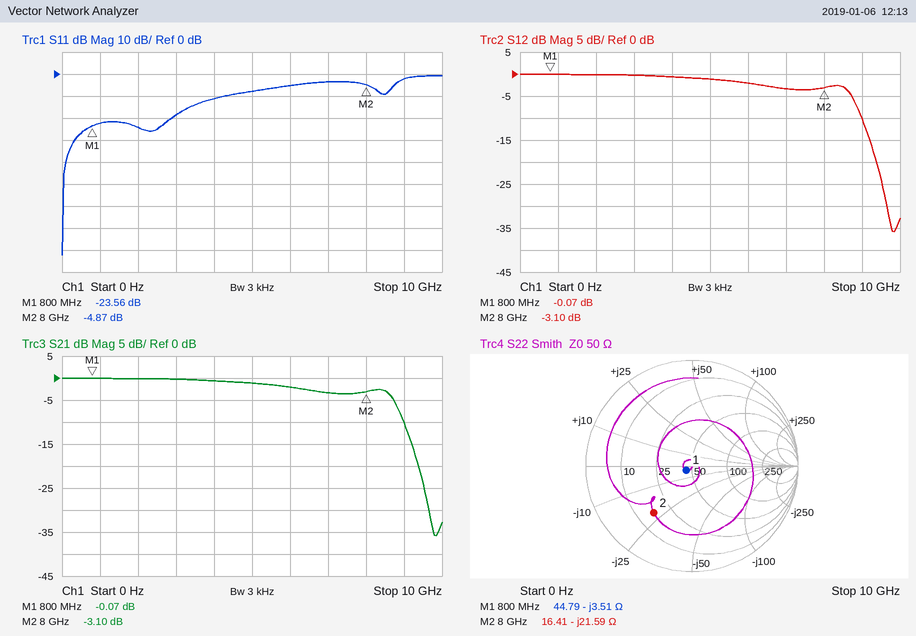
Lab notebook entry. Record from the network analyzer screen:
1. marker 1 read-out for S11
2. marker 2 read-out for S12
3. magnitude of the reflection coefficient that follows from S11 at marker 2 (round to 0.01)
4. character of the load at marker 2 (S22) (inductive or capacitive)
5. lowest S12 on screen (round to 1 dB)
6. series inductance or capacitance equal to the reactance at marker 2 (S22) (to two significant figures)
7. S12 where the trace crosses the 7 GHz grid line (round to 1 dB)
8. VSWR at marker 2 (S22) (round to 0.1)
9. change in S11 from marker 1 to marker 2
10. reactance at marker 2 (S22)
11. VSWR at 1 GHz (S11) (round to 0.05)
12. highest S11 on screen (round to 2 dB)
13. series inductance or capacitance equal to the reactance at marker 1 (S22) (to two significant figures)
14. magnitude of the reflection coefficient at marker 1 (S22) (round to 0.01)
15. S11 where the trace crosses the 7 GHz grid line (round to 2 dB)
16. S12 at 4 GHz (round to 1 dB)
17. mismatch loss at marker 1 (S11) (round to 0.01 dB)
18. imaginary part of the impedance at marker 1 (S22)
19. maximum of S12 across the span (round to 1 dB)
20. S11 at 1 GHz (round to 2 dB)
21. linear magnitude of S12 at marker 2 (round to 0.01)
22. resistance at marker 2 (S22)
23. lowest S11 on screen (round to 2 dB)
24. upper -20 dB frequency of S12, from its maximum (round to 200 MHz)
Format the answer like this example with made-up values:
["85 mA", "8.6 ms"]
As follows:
["-23.56 dB", "-3.10 dB", "0.57", "capacitive", "-36 dB", "920 fF", "-3 dB", "3.7", "18.69 dB", "-21.59 Ω", "1.15", "0 dB", "57 pF", "0.07", "-4 dB", "-1 dB", "0.02 dB", "-3.51 Ω", "0 dB", "-22 dB", "0.70", "16.41 Ω", "-82 dB", "9.4 GHz"]
